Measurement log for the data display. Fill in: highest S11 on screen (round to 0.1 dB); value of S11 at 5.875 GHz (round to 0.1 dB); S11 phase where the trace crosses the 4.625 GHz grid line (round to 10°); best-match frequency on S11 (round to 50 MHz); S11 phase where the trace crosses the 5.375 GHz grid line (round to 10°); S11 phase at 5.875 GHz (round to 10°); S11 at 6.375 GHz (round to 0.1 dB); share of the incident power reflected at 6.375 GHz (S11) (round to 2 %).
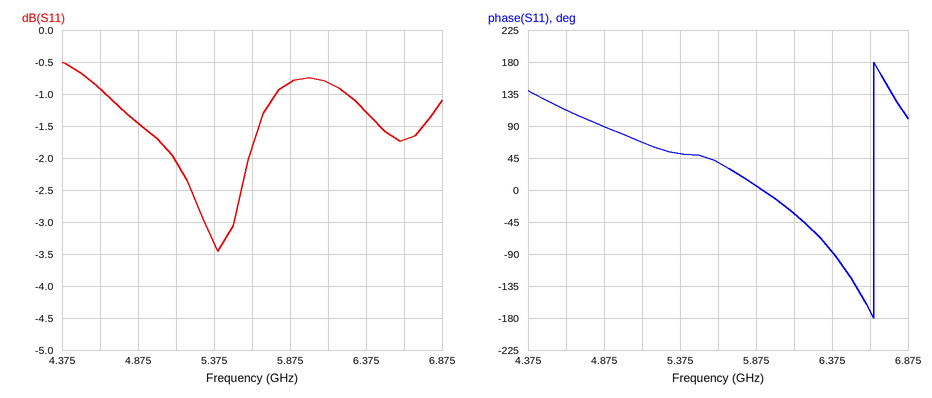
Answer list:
-0.5 dB
-0.8 dB
110°
5.40 GHz
50°
10°
-1.3 dB
74 %
